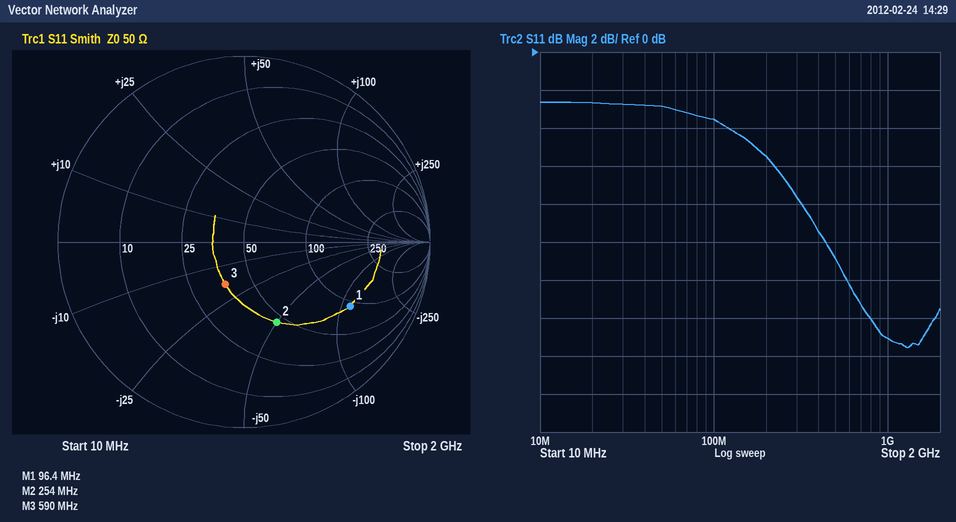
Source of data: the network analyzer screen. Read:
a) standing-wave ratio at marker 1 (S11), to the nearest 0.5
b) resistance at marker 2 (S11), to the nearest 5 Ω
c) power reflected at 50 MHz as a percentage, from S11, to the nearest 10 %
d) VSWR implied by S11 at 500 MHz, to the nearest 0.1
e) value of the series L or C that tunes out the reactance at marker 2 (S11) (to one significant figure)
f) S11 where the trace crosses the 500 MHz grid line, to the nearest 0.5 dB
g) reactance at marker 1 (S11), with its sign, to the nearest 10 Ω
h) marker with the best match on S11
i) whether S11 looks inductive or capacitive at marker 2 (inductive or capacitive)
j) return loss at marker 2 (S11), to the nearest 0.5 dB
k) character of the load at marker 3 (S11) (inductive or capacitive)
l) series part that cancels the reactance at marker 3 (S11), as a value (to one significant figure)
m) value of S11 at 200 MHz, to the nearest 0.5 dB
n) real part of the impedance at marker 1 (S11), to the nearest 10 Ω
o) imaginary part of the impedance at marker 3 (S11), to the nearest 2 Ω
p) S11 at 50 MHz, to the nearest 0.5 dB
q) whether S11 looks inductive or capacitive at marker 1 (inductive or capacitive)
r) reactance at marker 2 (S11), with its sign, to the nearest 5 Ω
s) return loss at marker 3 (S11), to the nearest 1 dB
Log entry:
5.0
45 Ω
50 %
1.8
30 nH
-11.0 dB
-110 Ω
marker 3
capacitive
6.5 dB
capacitive
5 nH
-5.5 dB
90 Ω
-18 Ω
-3.0 dB
capacitive
-50 Ω
12 dB
